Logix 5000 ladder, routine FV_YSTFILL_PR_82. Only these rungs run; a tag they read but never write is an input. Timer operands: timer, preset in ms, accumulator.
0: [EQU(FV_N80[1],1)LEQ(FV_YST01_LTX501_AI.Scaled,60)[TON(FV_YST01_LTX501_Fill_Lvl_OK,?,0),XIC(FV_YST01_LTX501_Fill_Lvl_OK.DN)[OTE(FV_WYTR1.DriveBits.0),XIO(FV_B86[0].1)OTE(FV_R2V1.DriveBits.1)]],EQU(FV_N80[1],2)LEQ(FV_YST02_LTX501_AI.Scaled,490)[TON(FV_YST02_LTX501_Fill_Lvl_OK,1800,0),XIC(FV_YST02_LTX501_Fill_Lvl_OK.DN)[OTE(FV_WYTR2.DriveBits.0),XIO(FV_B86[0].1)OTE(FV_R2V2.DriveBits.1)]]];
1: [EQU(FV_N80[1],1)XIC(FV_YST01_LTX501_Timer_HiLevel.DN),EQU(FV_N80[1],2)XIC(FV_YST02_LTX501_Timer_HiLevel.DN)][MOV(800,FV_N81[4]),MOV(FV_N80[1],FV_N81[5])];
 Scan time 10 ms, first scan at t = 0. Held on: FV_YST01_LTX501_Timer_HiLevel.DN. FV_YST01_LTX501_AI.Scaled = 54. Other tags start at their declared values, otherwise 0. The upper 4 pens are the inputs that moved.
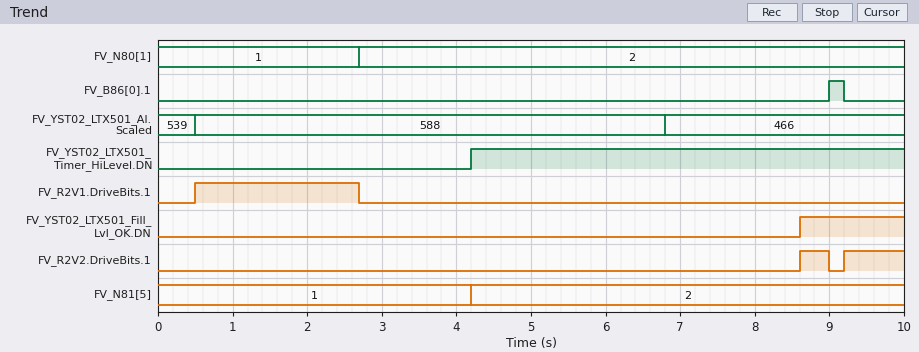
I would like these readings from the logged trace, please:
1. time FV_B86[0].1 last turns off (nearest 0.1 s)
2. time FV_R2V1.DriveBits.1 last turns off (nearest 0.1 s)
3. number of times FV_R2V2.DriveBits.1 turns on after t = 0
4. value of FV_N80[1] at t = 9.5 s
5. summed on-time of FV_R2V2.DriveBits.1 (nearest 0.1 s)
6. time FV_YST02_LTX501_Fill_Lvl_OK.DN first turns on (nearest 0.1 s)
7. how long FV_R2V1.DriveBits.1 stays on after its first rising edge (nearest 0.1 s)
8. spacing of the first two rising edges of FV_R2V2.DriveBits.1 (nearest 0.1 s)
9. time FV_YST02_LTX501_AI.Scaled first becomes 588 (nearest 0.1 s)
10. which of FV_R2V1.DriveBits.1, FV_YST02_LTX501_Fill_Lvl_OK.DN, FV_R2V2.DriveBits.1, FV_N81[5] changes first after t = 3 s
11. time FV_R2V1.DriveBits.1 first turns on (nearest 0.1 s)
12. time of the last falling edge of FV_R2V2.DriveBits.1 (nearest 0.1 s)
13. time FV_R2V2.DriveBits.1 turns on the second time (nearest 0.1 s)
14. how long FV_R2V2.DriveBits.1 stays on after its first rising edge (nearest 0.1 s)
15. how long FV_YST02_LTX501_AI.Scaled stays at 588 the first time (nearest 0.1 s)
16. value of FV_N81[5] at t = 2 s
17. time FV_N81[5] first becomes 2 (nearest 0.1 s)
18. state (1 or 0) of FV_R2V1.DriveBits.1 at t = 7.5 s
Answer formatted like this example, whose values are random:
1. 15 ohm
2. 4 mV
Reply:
1. 9.2 s
2. 2.7 s
3. 2
4. 2
5. 1.2 s
6. 8.6 s
7. 2.2 s
8. 0.6 s
9. 0.5 s
10. FV_N81[5]
11. 0.5 s
12. 9.0 s
13. 9.2 s
14. 0.4 s
15. 6.3 s
16. 1
17. 4.2 s
18. 0
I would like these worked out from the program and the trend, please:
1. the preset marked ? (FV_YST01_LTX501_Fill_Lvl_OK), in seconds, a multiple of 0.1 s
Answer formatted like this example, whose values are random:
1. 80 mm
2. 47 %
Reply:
1. 0.5 s
